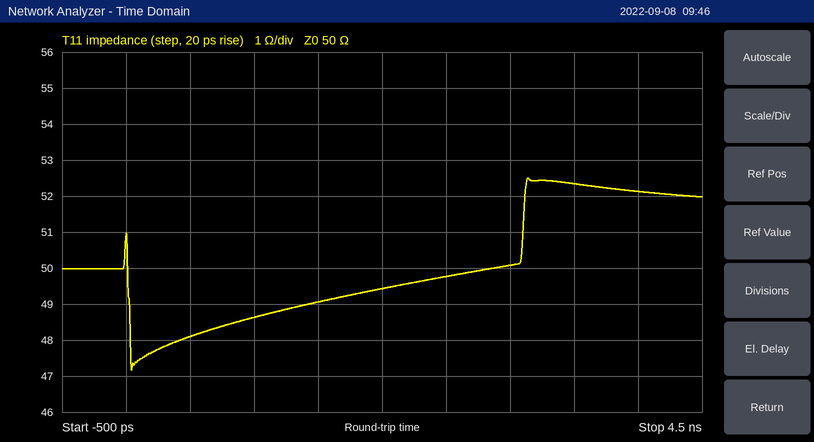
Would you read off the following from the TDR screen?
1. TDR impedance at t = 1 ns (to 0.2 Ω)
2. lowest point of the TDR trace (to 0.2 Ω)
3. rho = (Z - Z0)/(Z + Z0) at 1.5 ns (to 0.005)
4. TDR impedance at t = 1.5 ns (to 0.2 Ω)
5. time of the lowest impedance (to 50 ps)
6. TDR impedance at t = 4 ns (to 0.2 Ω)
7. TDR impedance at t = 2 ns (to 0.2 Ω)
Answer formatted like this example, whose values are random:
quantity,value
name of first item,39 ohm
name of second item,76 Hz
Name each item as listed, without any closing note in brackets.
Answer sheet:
quantity,value
TDR impedance at t = 1 ns,48.6 Ω
lowest point of the TDR trace,47.2 Ω
rho = (Z - Z0)/(Z + Z0) at 1.5 ns,-0.010
TDR impedance at t = 1.5 ns,49.0 Ω
time of the lowest impedance,50 ps
TDR impedance at t = 4 ns,52.2 Ω
TDR impedance at t = 2 ns,49.4 Ω
